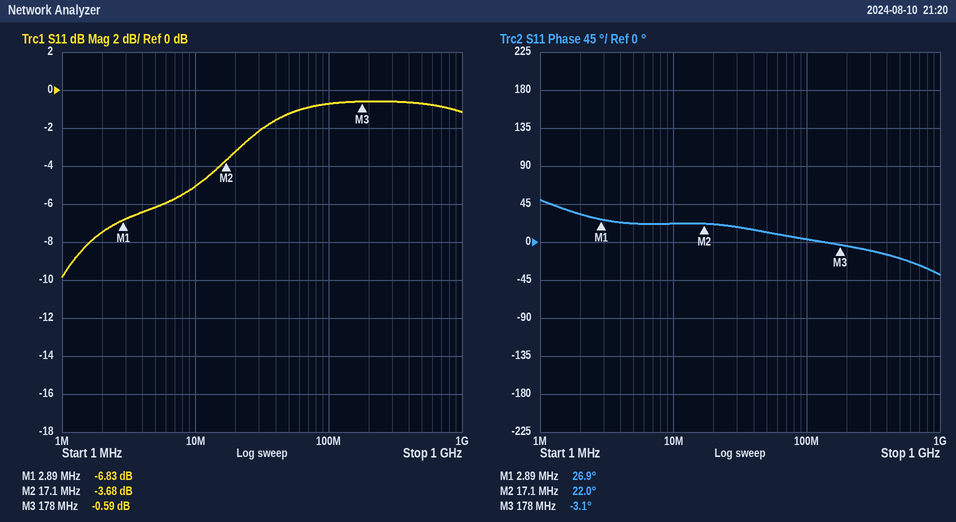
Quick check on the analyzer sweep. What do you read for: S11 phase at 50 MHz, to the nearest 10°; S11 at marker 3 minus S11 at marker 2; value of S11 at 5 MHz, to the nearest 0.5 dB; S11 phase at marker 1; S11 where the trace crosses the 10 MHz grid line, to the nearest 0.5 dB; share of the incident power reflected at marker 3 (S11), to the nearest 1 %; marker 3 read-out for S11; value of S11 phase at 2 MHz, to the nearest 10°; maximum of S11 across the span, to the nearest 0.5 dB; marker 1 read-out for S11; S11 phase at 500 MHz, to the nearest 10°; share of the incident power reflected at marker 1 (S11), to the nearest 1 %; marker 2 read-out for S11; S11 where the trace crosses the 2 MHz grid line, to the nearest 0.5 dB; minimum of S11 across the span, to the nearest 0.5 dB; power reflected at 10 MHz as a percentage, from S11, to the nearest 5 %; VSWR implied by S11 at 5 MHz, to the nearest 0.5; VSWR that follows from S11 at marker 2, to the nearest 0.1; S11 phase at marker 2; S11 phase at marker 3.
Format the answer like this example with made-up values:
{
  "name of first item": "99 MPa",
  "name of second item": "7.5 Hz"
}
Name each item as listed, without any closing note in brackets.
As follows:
{
  "S11 phase at 50 MHz, to the nearest 10°": "10°",
  "S11 at marker 3 minus S11 at marker 2": "3.09 dB",
  "value of S11 at 5 MHz, to the nearest 0.5 dB": "-6.0 dB",
  "S11 phase at marker 1": "26.9°",
  "S11 where the trace crosses the 10 MHz grid line, to the nearest 0.5 dB": "-5.0 dB",
  "share of the incident power reflected at marker 3 (S11), to the nearest 1 %": "87 %",
  "marker 3 read-out for S11": "-0.59 dB",
  "value of S11 phase at 2 MHz, to the nearest 10°": "30°",
  "maximum of S11 across the span, to the nearest 0.5 dB": "-0.5 dB",
  "marker 1 read-out for S11": "-6.83 dB",
  "S11 phase at 500 MHz, to the nearest 10°": "-20°",
  "share of the incident power reflected at marker 1 (S11), to the nearest 1 %": "21 %",
  "marker 2 read-out for S11": "-3.68 dB",
  "S11 where the trace crosses the 2 MHz grid line, to the nearest 0.5 dB": "-7.5 dB",
  "minimum of S11 across the span, to the nearest 0.5 dB": "-10.0 dB",
  "power reflected at 10 MHz as a percentage, from S11, to the nearest 5 %": "30 %",
  "VSWR implied by S11 at 5 MHz, to the nearest 0.5": "3.0",
  "VSWR that follows from S11 at marker 2, to the nearest 0.1": "4.8",
  "S11 phase at marker 2": "22.0°",
  "S11 phase at marker 3": "-3.1°"
}
